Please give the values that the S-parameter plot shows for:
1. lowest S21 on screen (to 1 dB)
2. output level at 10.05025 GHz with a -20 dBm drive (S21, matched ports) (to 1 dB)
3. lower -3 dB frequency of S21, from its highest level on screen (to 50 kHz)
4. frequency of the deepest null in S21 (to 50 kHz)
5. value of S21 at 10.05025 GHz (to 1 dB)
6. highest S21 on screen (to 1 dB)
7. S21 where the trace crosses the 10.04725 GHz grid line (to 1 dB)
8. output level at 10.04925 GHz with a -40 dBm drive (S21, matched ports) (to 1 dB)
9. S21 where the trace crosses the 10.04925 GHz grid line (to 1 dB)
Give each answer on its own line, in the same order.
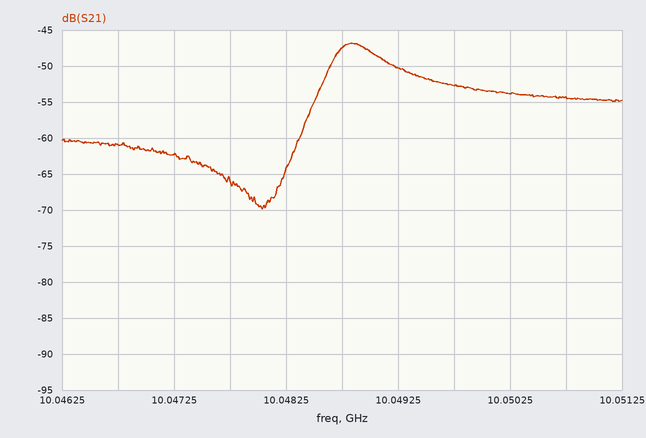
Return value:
-70 dB
-74 dBm
10.04865 GHz
10.04805 GHz
-54 dB
-47 dB
-62 dB
-90 dBm
-50 dB
